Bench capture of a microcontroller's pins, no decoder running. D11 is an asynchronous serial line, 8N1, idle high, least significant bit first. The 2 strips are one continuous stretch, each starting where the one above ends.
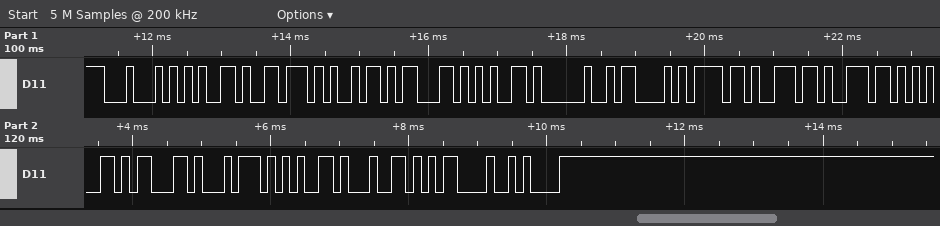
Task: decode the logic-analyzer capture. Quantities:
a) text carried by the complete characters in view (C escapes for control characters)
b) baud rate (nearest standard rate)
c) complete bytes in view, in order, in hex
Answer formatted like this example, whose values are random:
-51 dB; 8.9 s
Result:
"Device Connected\r\n"; 9600 baud; 44 65 76 69 63 65 20 43 6F 6E 6E 65 63 74 65 64 0D 0A
